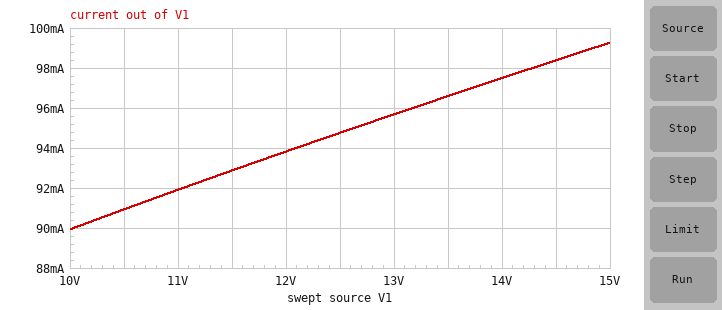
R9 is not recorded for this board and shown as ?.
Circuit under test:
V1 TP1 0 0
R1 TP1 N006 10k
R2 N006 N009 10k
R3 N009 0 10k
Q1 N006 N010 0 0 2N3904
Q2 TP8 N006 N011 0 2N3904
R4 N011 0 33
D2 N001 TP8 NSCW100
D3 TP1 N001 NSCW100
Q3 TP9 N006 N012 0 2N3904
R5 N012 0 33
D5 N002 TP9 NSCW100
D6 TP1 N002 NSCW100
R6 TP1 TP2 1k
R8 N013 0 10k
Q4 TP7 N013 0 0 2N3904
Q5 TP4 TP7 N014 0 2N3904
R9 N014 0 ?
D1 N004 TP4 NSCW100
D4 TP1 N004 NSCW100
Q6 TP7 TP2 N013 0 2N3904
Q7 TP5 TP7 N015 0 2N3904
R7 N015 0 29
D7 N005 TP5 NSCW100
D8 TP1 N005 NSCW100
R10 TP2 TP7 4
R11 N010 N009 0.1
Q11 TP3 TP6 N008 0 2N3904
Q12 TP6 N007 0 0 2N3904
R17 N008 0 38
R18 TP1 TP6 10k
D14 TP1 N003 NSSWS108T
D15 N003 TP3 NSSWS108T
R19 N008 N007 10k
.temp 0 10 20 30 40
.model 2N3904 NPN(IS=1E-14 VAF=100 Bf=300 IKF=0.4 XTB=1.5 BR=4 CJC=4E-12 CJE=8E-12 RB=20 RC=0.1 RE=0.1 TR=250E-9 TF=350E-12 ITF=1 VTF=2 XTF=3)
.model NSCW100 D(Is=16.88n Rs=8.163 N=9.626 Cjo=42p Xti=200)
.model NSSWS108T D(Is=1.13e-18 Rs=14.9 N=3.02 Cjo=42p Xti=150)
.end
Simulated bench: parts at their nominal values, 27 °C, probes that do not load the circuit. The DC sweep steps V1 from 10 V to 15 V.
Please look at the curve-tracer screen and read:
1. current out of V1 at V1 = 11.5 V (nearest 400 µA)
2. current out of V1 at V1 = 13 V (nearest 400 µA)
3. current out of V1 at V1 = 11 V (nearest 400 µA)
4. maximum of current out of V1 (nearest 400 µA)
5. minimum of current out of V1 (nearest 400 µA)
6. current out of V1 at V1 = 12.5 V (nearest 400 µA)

92.8 mA
95.6 mA
92.0 mA
99.2 mA
90.0 mA
94.8 mA
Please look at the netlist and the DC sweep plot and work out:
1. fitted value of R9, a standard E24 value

68 Ω
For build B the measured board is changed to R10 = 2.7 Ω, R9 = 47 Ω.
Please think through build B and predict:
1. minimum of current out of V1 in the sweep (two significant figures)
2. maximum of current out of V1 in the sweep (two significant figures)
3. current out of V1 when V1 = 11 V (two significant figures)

94 mA
100 mA
96 mA
